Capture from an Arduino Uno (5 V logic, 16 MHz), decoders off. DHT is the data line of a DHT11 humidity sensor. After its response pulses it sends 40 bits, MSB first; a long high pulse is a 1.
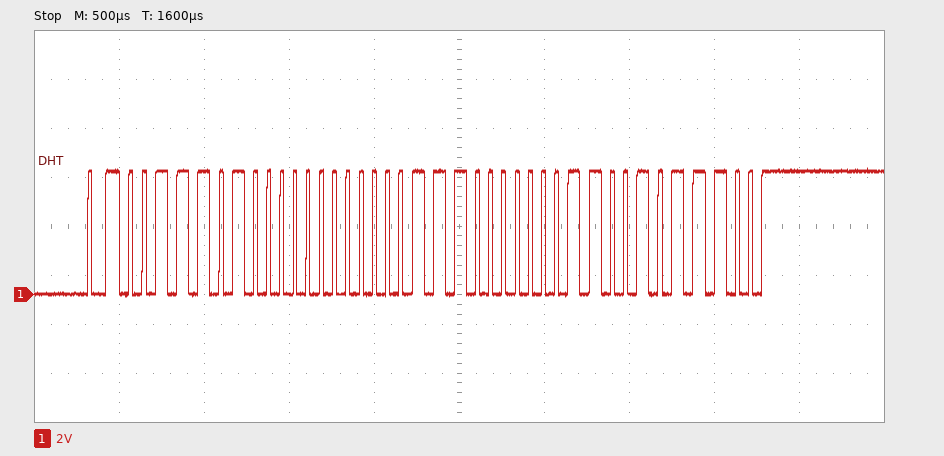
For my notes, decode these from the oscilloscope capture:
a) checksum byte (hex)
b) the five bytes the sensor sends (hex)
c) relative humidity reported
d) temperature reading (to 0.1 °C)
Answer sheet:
0x5C
3A 00 1C 06 5C
58 %
28.6 °C
